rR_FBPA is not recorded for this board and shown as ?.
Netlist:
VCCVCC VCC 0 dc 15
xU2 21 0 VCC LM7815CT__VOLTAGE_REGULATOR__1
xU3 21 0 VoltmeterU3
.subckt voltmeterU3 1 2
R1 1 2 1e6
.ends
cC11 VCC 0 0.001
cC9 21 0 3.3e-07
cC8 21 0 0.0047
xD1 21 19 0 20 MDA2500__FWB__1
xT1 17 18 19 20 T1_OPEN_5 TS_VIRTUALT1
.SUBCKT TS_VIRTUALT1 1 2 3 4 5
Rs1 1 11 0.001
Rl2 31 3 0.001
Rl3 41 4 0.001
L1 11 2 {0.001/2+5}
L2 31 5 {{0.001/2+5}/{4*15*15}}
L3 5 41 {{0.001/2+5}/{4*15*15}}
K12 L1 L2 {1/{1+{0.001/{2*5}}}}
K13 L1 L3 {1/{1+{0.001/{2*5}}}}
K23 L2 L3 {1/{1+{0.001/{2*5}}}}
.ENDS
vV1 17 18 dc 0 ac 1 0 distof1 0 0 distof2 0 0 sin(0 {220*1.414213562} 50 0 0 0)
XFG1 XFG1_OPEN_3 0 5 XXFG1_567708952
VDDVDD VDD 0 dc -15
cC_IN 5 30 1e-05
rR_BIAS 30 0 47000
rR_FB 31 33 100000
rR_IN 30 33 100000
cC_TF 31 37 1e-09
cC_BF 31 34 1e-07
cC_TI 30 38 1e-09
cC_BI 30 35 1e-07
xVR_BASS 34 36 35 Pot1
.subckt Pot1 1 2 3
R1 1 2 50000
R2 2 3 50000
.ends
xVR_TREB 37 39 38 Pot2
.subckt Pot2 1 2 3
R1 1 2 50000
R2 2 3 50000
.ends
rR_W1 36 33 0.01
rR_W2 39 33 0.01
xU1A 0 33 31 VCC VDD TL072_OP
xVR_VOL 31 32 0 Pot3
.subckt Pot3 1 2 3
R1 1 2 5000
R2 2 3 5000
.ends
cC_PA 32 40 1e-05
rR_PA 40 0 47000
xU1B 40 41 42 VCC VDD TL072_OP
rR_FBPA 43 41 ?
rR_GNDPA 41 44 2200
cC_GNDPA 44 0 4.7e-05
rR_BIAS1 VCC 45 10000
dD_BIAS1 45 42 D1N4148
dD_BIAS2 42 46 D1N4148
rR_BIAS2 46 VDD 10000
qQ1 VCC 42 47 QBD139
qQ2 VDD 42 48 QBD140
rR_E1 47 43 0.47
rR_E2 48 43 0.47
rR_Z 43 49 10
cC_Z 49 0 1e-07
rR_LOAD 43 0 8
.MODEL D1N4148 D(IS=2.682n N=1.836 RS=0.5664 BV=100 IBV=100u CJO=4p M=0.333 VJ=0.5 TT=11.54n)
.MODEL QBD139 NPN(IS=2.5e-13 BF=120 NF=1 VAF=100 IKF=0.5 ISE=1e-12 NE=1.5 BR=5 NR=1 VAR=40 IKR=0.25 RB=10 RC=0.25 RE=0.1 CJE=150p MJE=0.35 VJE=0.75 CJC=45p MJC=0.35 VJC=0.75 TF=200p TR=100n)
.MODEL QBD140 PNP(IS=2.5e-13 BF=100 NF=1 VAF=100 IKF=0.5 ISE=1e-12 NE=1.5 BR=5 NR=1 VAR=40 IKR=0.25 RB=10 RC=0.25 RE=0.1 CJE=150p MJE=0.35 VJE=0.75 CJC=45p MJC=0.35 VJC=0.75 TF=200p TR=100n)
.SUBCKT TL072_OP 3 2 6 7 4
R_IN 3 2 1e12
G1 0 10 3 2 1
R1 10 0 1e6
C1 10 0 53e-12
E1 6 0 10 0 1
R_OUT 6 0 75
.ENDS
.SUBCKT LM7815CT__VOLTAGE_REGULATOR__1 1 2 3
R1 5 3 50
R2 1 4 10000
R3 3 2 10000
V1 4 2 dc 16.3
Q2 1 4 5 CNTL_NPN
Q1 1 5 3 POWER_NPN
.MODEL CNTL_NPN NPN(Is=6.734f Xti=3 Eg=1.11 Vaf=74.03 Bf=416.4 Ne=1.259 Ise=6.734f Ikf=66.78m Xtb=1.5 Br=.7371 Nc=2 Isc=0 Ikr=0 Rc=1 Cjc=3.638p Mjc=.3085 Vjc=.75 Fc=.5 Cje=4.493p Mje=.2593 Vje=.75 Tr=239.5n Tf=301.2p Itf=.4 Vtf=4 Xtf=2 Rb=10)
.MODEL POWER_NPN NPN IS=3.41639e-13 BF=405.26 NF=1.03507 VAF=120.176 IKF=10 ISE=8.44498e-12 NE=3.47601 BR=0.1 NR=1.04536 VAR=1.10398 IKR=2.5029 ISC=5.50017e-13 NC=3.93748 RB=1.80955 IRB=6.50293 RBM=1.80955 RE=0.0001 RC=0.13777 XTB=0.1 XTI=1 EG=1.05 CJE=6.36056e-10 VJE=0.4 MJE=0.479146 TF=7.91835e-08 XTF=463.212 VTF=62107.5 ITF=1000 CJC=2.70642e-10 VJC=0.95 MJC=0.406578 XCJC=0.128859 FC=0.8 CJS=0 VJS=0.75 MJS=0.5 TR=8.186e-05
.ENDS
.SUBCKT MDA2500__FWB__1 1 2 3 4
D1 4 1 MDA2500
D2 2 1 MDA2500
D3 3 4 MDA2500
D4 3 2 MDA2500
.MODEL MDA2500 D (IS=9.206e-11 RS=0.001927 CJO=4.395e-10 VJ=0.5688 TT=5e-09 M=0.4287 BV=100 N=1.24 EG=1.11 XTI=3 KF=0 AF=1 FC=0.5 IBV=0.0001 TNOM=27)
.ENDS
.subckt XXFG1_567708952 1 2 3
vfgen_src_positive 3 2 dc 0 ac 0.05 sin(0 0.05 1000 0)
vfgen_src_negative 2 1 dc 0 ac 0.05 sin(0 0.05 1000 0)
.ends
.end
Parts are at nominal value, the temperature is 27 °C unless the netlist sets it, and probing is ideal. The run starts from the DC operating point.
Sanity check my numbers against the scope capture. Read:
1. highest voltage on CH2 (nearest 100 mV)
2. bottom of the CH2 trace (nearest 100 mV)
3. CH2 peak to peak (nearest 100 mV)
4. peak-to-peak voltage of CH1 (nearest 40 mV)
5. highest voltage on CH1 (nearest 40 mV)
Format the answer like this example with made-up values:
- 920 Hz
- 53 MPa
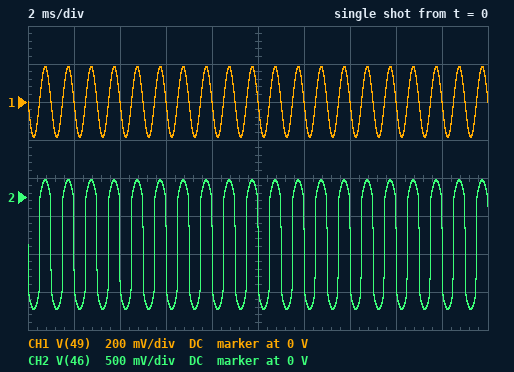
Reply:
- 200 mV
- -1.5 V
- 1.7 V
- 360 mV
- 200 mV
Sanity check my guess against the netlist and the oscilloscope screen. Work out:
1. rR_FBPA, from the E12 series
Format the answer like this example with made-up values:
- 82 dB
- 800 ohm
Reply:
- 15 kΩ
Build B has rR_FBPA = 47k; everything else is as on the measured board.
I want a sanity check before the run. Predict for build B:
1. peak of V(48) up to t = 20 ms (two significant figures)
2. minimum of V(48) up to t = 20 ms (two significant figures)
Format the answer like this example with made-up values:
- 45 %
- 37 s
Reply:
- 530 mV
- -560 mV
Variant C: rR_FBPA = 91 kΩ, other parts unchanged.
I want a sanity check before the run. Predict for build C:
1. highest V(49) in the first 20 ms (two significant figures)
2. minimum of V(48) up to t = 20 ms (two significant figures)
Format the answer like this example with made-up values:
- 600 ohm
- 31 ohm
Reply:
- 1.0 V
- -1.1 V
